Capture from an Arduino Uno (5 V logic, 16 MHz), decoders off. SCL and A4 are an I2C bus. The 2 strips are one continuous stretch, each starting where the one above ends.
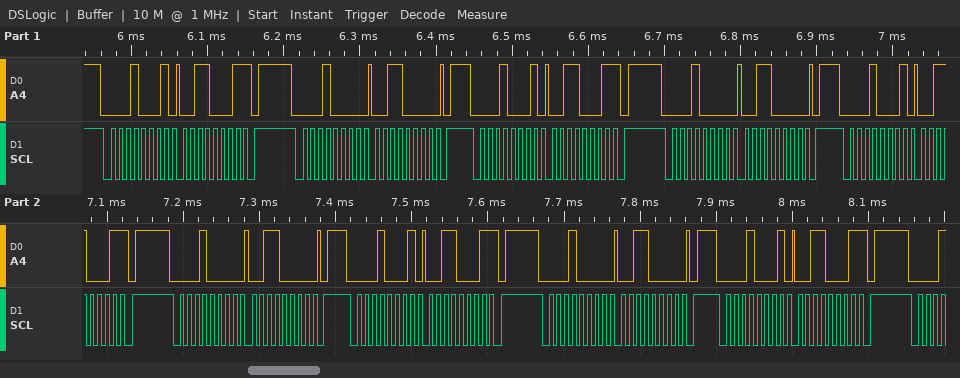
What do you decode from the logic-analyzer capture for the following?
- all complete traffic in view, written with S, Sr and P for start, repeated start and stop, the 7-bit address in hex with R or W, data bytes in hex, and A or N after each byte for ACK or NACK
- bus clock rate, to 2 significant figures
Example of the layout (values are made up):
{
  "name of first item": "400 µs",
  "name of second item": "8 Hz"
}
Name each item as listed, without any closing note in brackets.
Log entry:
{
  "all complete traffic in view, written with S, Sr and P for start, repeated start and stop, the 7-bit address in hex with R or W, data bytes in hex, and A or N after each byte for ACK or NACK": "S 08R A 31 N P S 08W A 30 A P S 08R A 31 N P S 08W A 30 A P S 08R A 31 N P S 08W A 30 A P S 08R A 31 N P S 08W A 30 A P S 08R A 31 N P",
  "bus clock rate, to 2 significant figures": "100 kHz"
}
